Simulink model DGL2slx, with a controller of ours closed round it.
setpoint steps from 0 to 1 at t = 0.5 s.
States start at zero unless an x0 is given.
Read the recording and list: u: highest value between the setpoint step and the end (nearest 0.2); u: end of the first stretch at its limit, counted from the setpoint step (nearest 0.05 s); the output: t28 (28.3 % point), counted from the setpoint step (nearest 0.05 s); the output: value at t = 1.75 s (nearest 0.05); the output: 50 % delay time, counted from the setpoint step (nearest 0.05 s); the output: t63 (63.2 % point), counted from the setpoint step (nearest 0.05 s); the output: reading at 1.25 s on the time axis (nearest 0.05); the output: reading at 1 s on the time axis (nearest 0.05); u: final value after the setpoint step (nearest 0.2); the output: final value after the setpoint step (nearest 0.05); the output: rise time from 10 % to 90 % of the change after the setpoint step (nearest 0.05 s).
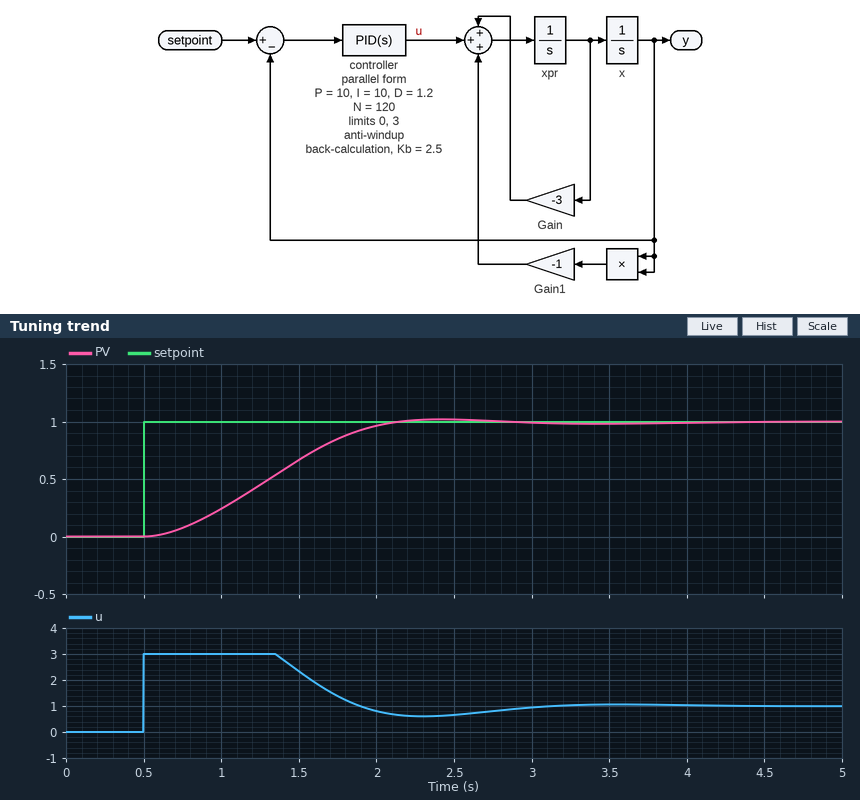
3.0
0.85 s
0.55 s
0.85
0.80 s
0.95 s
0.45
0.25
1.0
1.00
1.05 s
